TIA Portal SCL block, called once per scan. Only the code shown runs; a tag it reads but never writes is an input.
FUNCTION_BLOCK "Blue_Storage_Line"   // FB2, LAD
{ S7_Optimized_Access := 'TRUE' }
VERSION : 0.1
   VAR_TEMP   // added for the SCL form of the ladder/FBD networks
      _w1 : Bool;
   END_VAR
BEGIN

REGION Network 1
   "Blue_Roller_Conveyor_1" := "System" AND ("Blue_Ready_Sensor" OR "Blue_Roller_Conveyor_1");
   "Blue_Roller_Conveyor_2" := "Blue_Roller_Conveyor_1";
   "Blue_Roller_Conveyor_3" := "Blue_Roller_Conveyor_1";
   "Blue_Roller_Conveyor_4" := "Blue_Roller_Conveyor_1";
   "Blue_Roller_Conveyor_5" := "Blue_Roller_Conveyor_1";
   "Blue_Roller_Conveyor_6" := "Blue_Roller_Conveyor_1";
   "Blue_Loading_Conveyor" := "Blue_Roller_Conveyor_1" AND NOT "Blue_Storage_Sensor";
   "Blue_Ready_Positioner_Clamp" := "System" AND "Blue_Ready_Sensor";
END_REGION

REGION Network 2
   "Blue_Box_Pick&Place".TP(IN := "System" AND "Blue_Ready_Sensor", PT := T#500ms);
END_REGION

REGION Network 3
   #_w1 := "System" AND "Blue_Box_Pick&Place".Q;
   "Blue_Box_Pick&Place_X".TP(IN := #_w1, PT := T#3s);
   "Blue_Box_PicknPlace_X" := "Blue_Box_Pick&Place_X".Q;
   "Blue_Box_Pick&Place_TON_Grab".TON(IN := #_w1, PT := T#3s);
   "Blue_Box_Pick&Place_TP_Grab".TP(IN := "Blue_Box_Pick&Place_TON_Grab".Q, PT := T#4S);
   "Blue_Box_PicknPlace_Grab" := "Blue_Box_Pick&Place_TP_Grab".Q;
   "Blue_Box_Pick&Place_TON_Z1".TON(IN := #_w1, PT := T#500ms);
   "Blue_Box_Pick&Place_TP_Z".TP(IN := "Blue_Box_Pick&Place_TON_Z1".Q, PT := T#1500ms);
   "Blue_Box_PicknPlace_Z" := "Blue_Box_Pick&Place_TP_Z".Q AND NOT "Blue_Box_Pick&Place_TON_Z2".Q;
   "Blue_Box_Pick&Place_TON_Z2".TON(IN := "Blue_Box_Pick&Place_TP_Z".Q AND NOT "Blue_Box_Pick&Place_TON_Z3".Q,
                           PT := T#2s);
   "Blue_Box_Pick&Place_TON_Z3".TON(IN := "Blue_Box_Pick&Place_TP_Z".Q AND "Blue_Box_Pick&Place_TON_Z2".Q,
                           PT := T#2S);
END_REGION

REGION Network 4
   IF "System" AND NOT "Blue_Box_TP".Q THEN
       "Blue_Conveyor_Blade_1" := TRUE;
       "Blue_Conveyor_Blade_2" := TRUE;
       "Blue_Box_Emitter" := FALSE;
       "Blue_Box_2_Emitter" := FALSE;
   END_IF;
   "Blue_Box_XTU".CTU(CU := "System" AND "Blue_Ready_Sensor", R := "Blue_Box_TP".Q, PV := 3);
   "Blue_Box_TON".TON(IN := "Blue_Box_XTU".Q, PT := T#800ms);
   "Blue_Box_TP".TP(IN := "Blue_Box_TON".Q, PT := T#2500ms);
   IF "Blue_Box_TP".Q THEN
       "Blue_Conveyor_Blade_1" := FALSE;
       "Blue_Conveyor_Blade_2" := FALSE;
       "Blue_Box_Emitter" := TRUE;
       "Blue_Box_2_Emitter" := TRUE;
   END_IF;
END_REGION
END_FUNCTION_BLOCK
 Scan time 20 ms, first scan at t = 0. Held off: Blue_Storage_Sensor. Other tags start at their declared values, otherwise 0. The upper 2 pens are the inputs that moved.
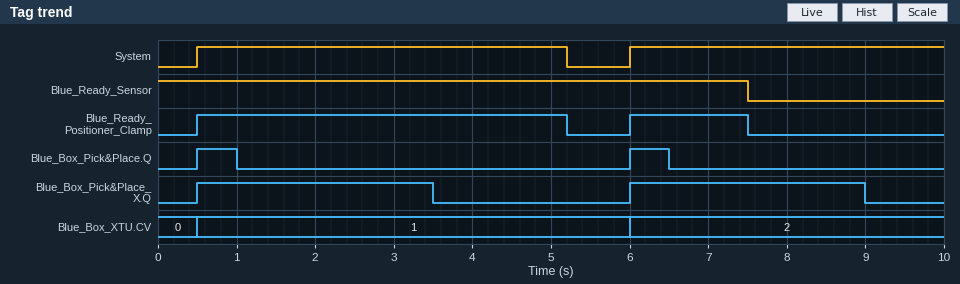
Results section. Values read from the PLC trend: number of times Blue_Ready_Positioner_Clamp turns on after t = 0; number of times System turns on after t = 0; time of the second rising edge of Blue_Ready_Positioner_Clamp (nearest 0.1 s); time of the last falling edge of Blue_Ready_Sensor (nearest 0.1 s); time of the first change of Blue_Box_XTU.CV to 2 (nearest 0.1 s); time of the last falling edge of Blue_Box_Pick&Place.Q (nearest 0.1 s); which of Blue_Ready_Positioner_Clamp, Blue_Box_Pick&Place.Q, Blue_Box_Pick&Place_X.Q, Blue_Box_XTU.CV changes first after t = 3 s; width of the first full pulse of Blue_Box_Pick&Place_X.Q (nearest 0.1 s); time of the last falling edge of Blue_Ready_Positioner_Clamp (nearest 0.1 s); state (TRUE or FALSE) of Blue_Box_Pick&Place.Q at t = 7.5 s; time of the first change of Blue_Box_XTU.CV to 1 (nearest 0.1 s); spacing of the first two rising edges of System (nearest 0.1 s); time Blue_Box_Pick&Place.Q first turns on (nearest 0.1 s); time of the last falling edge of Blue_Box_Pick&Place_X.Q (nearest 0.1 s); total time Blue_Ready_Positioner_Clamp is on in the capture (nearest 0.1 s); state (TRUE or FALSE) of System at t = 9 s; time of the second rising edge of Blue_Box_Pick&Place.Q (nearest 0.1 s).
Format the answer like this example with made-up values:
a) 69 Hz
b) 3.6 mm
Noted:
a) 2
b) 2
c) 6.0 s
d) 7.5 s
e) 6.0 s
f) 6.5 s
g) Blue_Box_Pick&Place_X.Q
h) 3.0 s
i) 7.5 s
j) FALSE
k) 0.5 s
l) 5.5 s
m) 0.5 s
n) 9.0 s
o) 6.2 s
p) TRUE
q) 6.0 s
